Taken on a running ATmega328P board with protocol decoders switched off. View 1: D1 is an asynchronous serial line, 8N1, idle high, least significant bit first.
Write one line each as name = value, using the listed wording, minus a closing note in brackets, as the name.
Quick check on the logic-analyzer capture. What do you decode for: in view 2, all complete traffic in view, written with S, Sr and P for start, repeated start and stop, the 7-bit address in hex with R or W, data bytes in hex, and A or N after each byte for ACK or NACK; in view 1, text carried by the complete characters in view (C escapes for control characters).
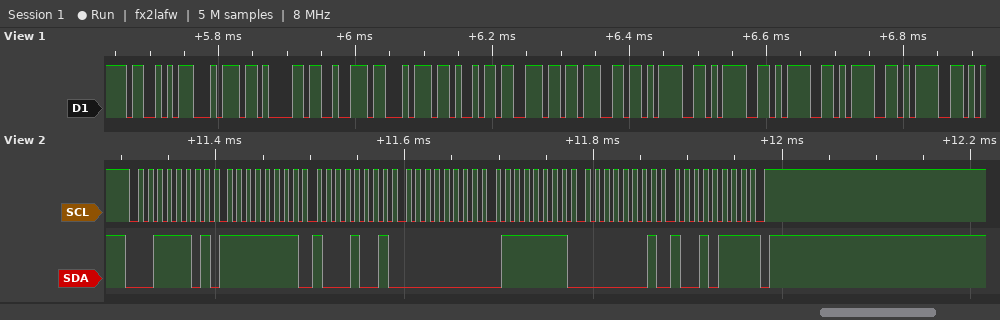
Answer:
in view 2, all complete traffic in view, written with S, Sr and P for start, repeated start and stop, the 7-bit address in hex with R or W, data bytes in hex, and A or N after each byte for ACK or NACK = S 1ER A FF A 89 A 00 A 7F A 01 A 97 N P
in view 1, text carried by the complete characters in view = "Starting====="
